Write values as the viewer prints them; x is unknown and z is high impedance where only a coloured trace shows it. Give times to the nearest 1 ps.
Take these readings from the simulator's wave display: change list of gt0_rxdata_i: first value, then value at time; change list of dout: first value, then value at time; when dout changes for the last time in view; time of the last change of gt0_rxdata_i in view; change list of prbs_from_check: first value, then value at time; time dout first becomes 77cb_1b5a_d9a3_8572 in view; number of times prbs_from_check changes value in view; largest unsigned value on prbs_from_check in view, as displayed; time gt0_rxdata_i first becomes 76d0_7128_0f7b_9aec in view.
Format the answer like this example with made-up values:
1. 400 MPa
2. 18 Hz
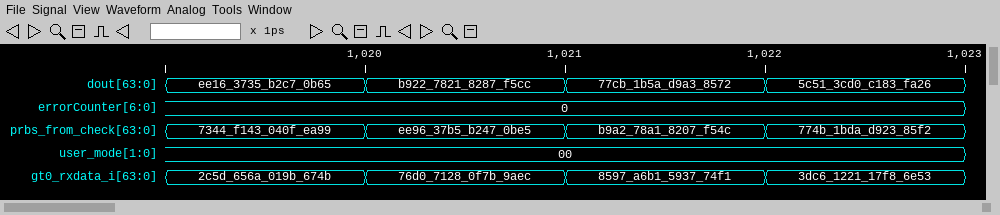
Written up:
1. 2c5d_656a_019b_674b, 76d0_7128_0f7b_9aec at 1020 ps, 8597_a6b1_5937_74f1 at 1021 ps, 3dc6_1221_17f8_6e53 at 1022 ps
2. ee16_3735_b2c7_0b65, b922_7821_8287_f5cc at 1020 ps, 77cb_1b5a_d9a3_8572 at 1021 ps, 5c51_3cd0_c183_fa26 at 1022 ps
3. 1022 ps
4. 1022 ps
5. 7344_f143_040f_ea99, ee96_37b5_b247_0be5 at 1020 ps, b9a2_78a1_8207_f54c at 1021 ps, 774b_1bda_d923_85f2 at 1022 ps
6. 1021 ps
7. 3
8. ee96_37b5_b247_0be5
9. 1020 ps
